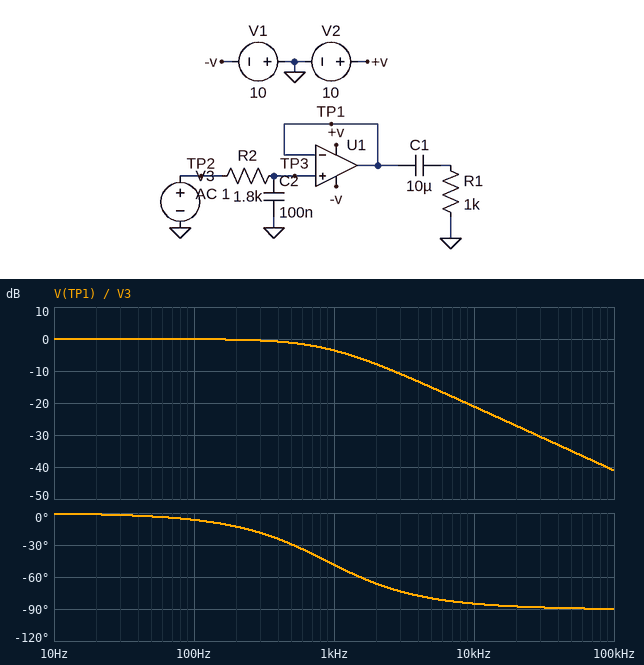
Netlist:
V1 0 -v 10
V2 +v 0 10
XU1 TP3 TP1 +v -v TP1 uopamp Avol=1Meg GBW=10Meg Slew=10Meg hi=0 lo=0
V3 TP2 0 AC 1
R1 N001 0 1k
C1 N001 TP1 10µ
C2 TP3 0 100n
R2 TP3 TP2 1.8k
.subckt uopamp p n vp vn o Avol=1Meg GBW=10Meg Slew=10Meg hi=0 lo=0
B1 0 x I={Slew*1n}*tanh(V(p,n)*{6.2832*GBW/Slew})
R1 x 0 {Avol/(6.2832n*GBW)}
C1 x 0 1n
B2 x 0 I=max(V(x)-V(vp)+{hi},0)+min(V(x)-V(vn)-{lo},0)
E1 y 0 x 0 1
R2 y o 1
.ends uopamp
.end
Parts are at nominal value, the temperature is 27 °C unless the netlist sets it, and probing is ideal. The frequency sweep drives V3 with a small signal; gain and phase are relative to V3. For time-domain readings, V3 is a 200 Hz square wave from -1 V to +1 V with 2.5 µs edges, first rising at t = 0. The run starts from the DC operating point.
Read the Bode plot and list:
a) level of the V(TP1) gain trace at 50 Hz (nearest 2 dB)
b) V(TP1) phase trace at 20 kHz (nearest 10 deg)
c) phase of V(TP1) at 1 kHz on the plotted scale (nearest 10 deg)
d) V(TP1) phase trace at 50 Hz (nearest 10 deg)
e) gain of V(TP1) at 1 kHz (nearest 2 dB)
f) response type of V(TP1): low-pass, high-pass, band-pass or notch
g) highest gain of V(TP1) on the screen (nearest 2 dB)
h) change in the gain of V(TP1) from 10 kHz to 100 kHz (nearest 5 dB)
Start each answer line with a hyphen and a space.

- 0 dB
- -90 deg
- -50 deg
- 0 deg
- -4 dB
- low-pass
- 0 dB
- -20 dB
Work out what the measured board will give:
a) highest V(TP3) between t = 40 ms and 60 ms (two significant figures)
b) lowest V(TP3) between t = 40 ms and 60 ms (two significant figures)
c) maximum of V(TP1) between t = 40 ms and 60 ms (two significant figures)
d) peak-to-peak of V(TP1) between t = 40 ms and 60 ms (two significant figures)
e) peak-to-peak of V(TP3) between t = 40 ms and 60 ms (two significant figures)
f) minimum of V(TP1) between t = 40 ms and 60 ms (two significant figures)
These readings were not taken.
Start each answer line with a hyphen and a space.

- 1.0 V
- -1.0 V
- 1.0 V
- 2.0 V
- 2.0 V
- -1.0 V
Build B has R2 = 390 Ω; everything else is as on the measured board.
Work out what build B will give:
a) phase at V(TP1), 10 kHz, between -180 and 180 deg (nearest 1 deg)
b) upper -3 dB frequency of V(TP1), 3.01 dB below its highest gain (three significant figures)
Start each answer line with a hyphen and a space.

- -68 deg
- 4.08 kHz
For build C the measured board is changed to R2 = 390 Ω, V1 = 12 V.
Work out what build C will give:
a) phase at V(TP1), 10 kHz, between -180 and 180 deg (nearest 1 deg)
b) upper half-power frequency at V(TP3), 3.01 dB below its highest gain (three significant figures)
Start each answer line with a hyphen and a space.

- -68 deg
- 4.08 kHz
